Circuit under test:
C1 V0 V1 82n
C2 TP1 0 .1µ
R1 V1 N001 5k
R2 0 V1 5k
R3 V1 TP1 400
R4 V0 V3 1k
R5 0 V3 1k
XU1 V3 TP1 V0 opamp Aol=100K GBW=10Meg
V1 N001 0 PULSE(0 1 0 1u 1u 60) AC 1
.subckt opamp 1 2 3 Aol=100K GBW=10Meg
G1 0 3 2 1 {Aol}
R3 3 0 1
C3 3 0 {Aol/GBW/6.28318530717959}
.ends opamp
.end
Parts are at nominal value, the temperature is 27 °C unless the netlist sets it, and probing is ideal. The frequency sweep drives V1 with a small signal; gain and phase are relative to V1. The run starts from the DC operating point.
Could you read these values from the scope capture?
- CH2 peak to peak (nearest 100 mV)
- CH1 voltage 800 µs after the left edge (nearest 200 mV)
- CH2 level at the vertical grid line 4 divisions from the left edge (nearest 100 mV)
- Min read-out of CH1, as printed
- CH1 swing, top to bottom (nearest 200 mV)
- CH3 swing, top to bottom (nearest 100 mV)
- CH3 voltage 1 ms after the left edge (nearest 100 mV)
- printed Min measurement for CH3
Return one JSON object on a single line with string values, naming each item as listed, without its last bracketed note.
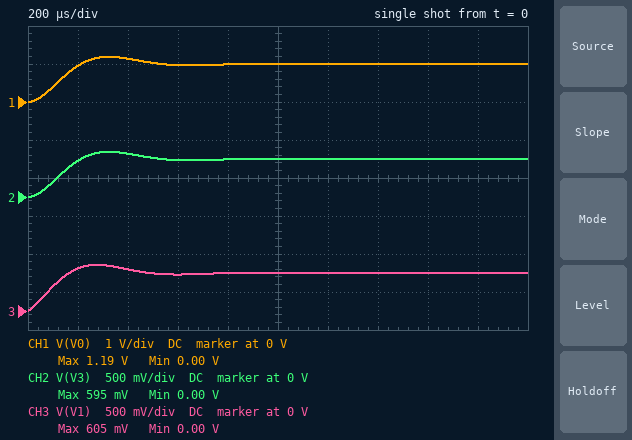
{"CH2 peak to peak": "600 mV", "CH1 voltage 800 µs after the left edge": "1.0 V", "CH2 level at the vertical grid line 4 divisions from the left edge": "500 mV", "Min read-out of CH1, as printed": "0.00 V", "CH1 swing, top to bottom": "1.2 V", "CH3 swing, top to bottom": "600 mV", "CH3 voltage 1 ms after the left edge": "500 mV", "printed Min measurement for CH3": "0.00 V"}
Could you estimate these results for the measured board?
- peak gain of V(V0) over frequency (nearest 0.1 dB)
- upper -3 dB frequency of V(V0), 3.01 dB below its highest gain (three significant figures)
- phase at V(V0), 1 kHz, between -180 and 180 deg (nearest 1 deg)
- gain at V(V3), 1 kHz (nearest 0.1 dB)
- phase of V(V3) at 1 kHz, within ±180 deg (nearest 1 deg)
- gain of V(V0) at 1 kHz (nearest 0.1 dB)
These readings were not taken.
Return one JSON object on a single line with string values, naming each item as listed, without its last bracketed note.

{"peak gain of V(V0) over frequency": "1.6 dB", "upper -3 dB frequency of V(V0), 3.01 dB below its highest gain": "2.07 kHz", "phase at V(V0), 1 kHz, between -180 and 180 deg": "-38 deg", "gain at V(V3), 1 kHz": "-4.7 dB", "phase of V(V3) at 1 kHz, within ±180 deg": "-38 deg", "gain of V(V0) at 1 kHz": "1.3 dB"}
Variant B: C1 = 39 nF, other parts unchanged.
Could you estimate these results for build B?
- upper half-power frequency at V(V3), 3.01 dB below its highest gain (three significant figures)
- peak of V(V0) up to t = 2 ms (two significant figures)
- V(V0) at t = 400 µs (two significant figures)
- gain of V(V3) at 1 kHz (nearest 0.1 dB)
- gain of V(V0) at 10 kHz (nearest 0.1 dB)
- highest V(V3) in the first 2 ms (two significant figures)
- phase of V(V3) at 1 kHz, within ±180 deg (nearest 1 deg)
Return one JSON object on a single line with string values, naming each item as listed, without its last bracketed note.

{"upper half-power frequency at V(V3), 3.01 dB below its highest gain": "923 Hz", "peak of V(V0) up to t = 2 ms": "1.0 V", "V(V0) at t = 400 µs": "890 mV", "gain of V(V3) at 1 kHz": "-9.4 dB", "gain of V(V0) at 10 kHz": "-25.5 dB", "highest V(V3) in the first 2 ms": "500 mV", "phase of V(V3) at 1 kHz, within ±180 deg": "-55 deg"}
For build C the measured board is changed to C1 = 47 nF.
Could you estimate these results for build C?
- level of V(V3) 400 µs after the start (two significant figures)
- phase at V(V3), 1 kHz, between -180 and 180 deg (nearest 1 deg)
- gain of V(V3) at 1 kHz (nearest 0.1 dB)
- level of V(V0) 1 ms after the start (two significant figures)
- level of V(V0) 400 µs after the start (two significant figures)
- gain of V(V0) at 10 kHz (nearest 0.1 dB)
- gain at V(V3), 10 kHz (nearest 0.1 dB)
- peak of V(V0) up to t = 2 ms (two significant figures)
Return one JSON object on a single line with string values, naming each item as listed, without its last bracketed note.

{"level of V(V3) 400 µs after the start": "460 mV", "phase at V(V3), 1 kHz, between -180 and 180 deg": "-53 deg", "gain of V(V3) at 1 kHz": "-8.7 dB", "level of V(V0) 1 ms after the start": "1.0 V", "level of V(V0) 400 µs after the start": "930 mV", "gain of V(V0) at 10 kHz": "-26.3 dB", "gain at V(V3), 10 kHz": "-32.3 dB", "peak of V(V0) up to t = 2 ms": "1.0 V"}
